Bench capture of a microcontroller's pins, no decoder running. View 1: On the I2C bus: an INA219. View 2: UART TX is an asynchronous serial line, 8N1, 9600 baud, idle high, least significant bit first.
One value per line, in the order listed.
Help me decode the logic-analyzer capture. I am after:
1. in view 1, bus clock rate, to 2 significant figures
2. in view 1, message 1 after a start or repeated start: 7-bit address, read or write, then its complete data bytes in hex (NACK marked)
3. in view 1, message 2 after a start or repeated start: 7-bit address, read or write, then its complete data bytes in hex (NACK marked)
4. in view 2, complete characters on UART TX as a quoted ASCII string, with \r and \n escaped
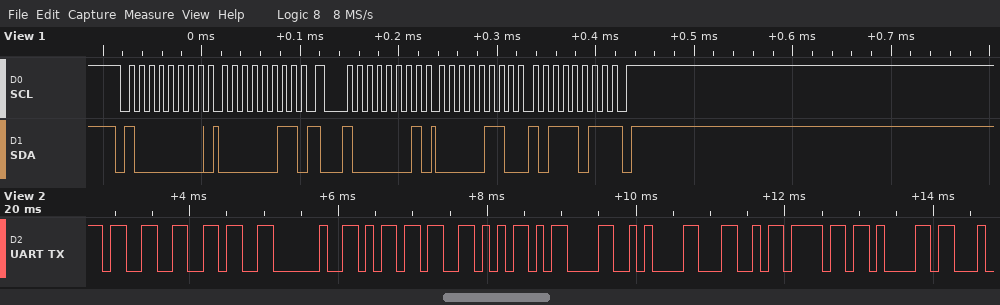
100 kHz
0x40 write: 03
0x40 read: 06 BB NACK
"36 mV\r\nLoa"
